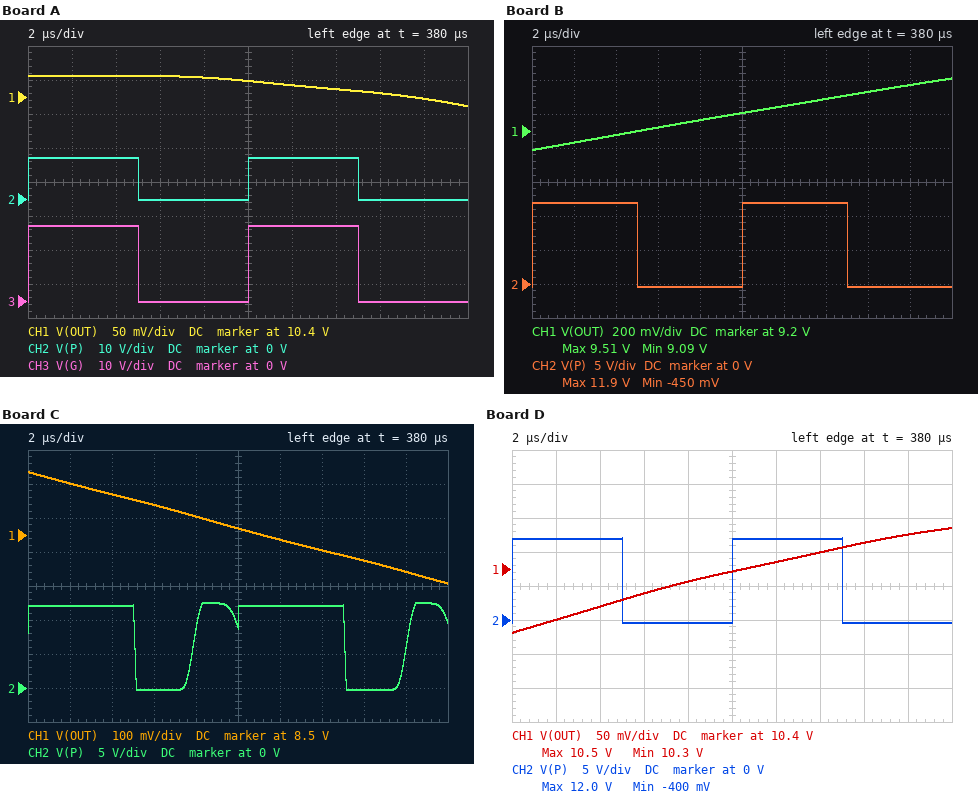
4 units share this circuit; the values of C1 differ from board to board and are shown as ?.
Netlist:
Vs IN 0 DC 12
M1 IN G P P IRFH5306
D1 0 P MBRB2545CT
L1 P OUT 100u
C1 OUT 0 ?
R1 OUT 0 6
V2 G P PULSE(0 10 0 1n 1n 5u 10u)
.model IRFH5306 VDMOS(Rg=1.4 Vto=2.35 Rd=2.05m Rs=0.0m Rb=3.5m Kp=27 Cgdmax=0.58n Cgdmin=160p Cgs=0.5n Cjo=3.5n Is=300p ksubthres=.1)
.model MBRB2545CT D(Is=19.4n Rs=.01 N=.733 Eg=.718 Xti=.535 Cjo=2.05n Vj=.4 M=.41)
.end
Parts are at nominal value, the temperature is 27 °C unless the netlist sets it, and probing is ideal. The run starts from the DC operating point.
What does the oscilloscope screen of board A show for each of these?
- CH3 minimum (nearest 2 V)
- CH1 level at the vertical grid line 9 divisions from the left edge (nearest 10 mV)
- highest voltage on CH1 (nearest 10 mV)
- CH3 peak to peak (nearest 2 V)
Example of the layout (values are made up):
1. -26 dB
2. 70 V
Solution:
1. 0 V
2. 10.40 V
3. 10.43 V
4. 22 V
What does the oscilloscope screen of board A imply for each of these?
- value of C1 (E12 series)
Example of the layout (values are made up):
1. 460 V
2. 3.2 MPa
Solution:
1. 150 µF
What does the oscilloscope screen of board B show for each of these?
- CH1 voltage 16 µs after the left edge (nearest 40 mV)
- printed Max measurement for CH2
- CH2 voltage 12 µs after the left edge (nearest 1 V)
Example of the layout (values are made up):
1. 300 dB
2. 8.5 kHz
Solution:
1. 9.44 V
2. 11.9 V
3. 12 V
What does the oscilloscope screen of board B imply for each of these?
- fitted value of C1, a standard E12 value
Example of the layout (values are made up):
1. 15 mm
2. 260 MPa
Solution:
1. 270 µF
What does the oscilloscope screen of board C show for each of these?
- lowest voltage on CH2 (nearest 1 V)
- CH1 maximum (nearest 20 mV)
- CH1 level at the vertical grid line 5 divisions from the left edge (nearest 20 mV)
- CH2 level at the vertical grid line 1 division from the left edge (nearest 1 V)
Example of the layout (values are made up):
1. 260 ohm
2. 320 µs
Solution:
1. 0 V
2. 8.68 V
3. 8.52 V
4. 12 V
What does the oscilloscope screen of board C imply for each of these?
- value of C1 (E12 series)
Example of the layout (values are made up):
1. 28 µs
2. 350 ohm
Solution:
1. 82 µF
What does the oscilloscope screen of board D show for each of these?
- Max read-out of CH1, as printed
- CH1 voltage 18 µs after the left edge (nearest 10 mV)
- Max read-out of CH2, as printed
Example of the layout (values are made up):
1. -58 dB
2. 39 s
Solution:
1. 10.5 V
2. 10.45 V
3. 12.0 V
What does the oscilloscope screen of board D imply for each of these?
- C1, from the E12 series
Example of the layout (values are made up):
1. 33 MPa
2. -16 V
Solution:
1. 180 µF
